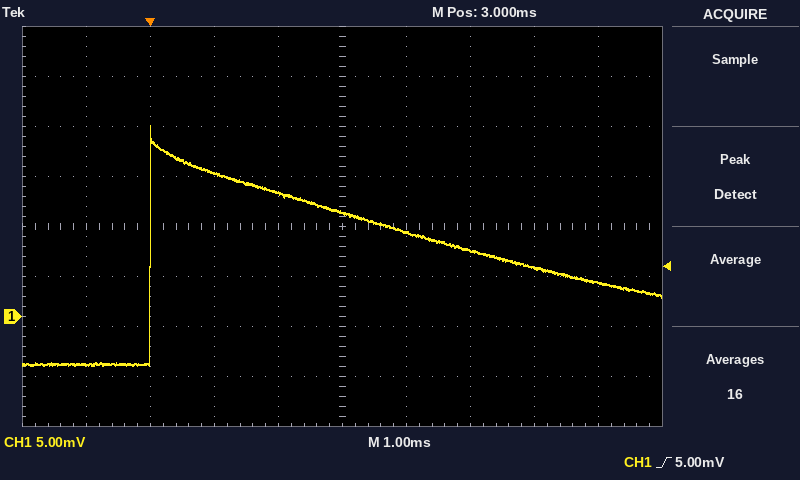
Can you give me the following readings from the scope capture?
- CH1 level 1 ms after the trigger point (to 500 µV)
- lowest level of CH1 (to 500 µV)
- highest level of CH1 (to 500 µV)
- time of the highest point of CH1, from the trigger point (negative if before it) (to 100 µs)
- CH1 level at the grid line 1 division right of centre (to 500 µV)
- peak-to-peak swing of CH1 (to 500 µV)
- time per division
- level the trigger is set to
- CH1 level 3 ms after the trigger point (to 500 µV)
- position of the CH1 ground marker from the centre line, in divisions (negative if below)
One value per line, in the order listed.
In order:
14.5 mV
-5.0 mV
19.0 mV
0.0 ms
8.5 mV
24.0 mV
1 ms
5.00 mV
10.5 mV
-1.8 div
